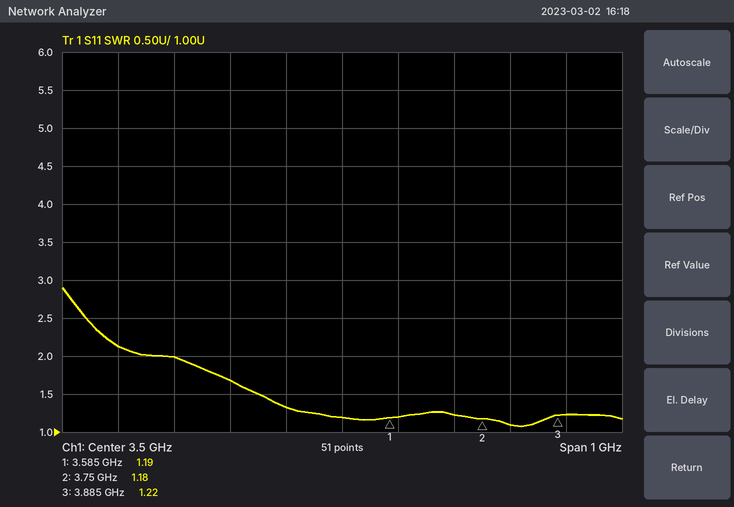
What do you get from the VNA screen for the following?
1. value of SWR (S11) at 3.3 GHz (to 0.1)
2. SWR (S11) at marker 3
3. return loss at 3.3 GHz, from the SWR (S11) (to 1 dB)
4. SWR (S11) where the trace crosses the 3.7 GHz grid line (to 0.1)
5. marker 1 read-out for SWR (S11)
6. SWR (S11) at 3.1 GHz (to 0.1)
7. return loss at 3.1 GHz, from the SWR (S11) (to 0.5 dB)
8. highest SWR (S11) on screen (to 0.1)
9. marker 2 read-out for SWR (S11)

1.7
1.22
12 dB
1.2
1.19
2.1
9.0 dB
2.9
1.18
